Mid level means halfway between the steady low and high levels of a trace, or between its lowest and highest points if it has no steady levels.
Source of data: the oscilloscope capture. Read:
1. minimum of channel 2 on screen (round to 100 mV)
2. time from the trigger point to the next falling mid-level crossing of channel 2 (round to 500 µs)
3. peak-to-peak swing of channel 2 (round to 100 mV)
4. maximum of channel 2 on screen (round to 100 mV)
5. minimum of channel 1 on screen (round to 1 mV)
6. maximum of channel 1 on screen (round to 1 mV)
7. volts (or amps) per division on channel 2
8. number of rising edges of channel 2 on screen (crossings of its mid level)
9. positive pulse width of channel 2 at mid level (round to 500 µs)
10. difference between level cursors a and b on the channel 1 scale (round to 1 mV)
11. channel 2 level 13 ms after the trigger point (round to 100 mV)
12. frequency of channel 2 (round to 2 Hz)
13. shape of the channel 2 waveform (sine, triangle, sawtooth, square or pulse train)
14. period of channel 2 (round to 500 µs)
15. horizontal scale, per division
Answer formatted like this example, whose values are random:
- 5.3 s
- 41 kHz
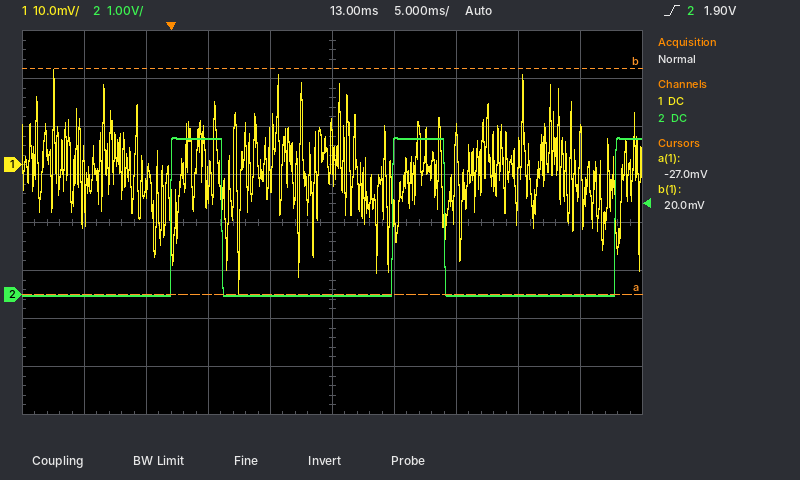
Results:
- 0.0 V
- 4.0 ms
- 3.3 V
- 3.3 V
- -27 mV
- 20 mV
- 1 V
- 3
- 4.0 ms
- 47 mV
- 0.0 V
- 56 Hz
- pulse train
- 18.0 ms
- 5 ms
